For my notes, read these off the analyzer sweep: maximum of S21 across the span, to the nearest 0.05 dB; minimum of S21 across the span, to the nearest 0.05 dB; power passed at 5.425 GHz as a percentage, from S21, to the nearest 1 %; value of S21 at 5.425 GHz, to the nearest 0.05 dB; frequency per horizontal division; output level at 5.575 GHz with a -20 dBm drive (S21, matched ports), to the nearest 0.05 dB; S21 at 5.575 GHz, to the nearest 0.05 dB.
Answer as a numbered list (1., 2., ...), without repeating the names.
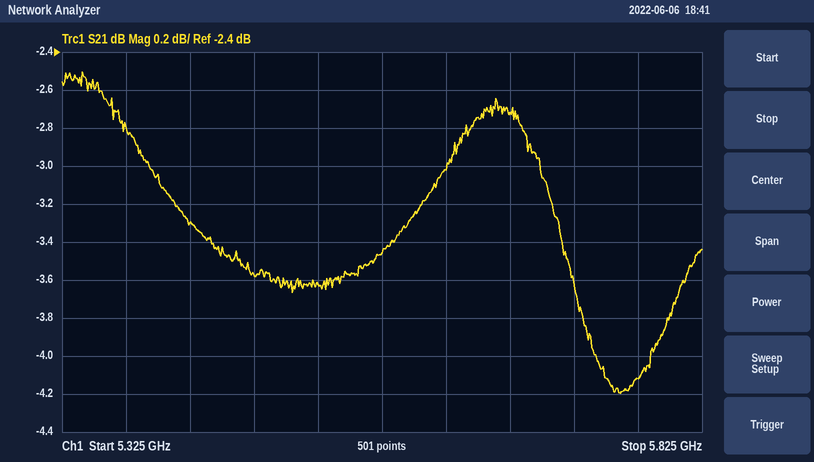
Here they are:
1. -2.50 dB
2. -4.20 dB
3. 47 %
4. -3.30 dB
5. 50 MHz
6. -23.45 dBm
7. -3.45 dB
